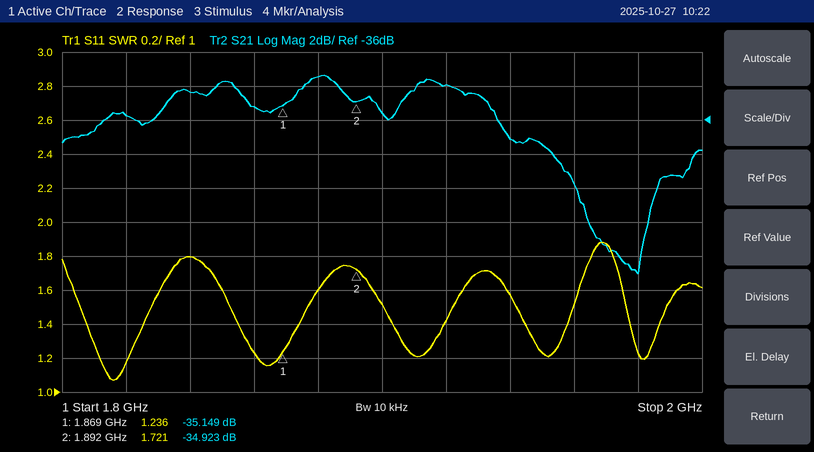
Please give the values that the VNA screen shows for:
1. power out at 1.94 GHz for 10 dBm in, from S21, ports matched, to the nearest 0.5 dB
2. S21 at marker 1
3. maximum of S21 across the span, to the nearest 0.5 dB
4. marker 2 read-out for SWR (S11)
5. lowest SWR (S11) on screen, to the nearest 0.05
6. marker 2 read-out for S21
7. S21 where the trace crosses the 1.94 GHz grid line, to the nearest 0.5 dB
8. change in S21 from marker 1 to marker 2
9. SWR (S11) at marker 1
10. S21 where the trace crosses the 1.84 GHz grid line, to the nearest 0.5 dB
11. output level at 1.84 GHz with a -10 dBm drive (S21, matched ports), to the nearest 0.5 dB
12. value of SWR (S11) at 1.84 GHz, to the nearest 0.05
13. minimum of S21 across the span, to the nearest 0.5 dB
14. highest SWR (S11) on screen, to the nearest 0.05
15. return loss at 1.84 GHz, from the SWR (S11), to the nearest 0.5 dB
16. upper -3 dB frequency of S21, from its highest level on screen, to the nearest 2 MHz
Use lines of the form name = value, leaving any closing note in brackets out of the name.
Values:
power out at 1.94 GHz for 10 dBm in, from S21, ports matched, to the nearest 0.5 dB = -27.0 dBm
S21 at marker 1 = -35.149 dB
maximum of S21 across the span, to the nearest 0.5 dB = -33.5 dB
marker 2 read-out for SWR = 1.721
lowest SWR (S11) on screen, to the nearest 0.05 = 1.05
marker 2 read-out for S21 = -34.923 dB
S21 where the trace crosses the 1.94 GHz grid line, to the nearest 0.5 dB = -37.0 dB
change in S21 from marker 1 to marker 2 = 0.226 dB
SWR (S11) at marker 1 = 1.236
S21 where the trace crosses the 1.84 GHz grid line, to the nearest 0.5 dB = -34.5 dB
output level at 1.84 GHz with a -10 dBm drive (S21, matched ports), to the nearest 0.5 dB = -44.5 dBm
value of SWR (S11) at 1.84 GHz, to the nearest 0.05 = 1.80
minimum of S21 across the span, to the nearest 0.5 dB = -45.0 dB
highest SWR (S11) on screen, to the nearest 0.05 = 1.90
return loss at 1.84 GHz, from the SWR (S11), to the nearest 0.5 dB = 11.0 dB
upper -3 dB frequency of S21, from its highest level on screen, to the nearest 2 MHz = 1.938 GHz
